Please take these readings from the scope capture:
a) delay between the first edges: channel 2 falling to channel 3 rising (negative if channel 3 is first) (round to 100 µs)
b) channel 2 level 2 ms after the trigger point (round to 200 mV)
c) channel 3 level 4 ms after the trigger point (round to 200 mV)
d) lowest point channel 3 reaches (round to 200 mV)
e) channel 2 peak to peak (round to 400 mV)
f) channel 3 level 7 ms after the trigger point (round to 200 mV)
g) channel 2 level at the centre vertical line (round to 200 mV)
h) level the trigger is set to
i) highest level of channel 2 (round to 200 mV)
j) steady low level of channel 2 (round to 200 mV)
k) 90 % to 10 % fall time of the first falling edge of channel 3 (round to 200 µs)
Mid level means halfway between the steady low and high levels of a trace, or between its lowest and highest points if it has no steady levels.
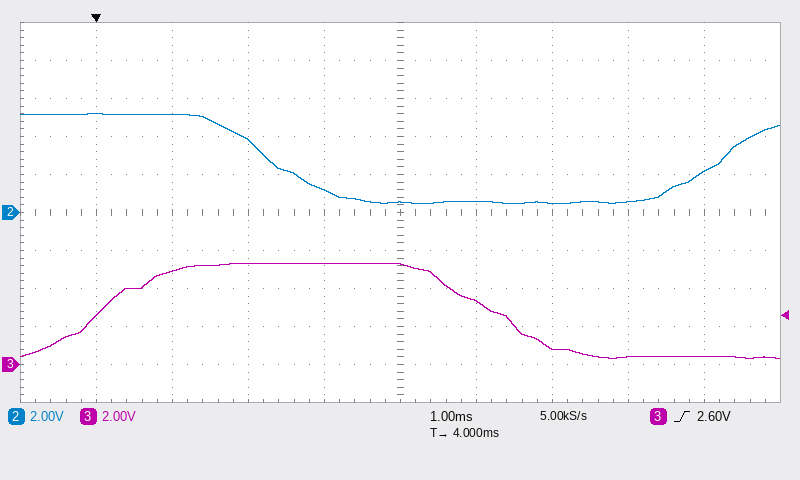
-2.2 ms
3.8 V
5.2 V
400 mV
4.8 V
400 mV
600 mV
2.60 V
5.2 V
600 mV
1.6 ms
